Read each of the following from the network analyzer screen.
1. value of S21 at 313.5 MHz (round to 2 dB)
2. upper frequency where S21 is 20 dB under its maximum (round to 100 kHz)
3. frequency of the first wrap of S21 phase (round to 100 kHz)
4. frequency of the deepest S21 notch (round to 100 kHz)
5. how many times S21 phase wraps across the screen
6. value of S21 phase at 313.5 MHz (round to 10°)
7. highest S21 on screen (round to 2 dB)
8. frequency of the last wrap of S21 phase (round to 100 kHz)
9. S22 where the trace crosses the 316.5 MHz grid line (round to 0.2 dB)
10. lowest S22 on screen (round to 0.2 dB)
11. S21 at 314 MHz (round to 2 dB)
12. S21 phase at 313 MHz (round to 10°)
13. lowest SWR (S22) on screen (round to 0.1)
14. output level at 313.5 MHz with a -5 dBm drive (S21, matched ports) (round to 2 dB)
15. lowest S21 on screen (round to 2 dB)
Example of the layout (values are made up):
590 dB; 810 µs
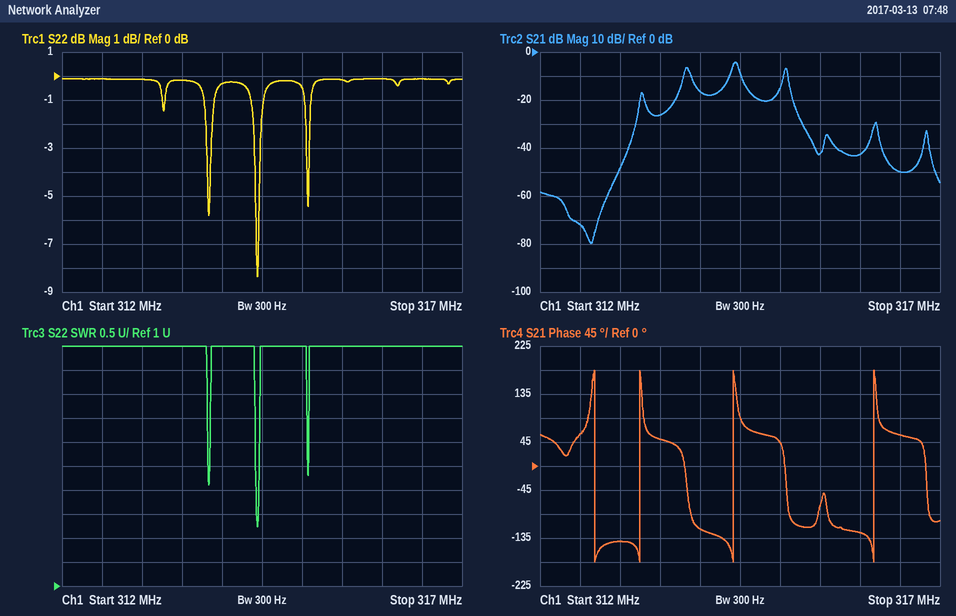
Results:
-26 dB; 315.2 MHz; 312.7 MHz; 312.6 MHz; 4; 50°; -4 dB; 316.2 MHz; -0.2 dB; -8.4 dB; -16 dB; -140°; 2.2; -32 dBm; -80 dB
